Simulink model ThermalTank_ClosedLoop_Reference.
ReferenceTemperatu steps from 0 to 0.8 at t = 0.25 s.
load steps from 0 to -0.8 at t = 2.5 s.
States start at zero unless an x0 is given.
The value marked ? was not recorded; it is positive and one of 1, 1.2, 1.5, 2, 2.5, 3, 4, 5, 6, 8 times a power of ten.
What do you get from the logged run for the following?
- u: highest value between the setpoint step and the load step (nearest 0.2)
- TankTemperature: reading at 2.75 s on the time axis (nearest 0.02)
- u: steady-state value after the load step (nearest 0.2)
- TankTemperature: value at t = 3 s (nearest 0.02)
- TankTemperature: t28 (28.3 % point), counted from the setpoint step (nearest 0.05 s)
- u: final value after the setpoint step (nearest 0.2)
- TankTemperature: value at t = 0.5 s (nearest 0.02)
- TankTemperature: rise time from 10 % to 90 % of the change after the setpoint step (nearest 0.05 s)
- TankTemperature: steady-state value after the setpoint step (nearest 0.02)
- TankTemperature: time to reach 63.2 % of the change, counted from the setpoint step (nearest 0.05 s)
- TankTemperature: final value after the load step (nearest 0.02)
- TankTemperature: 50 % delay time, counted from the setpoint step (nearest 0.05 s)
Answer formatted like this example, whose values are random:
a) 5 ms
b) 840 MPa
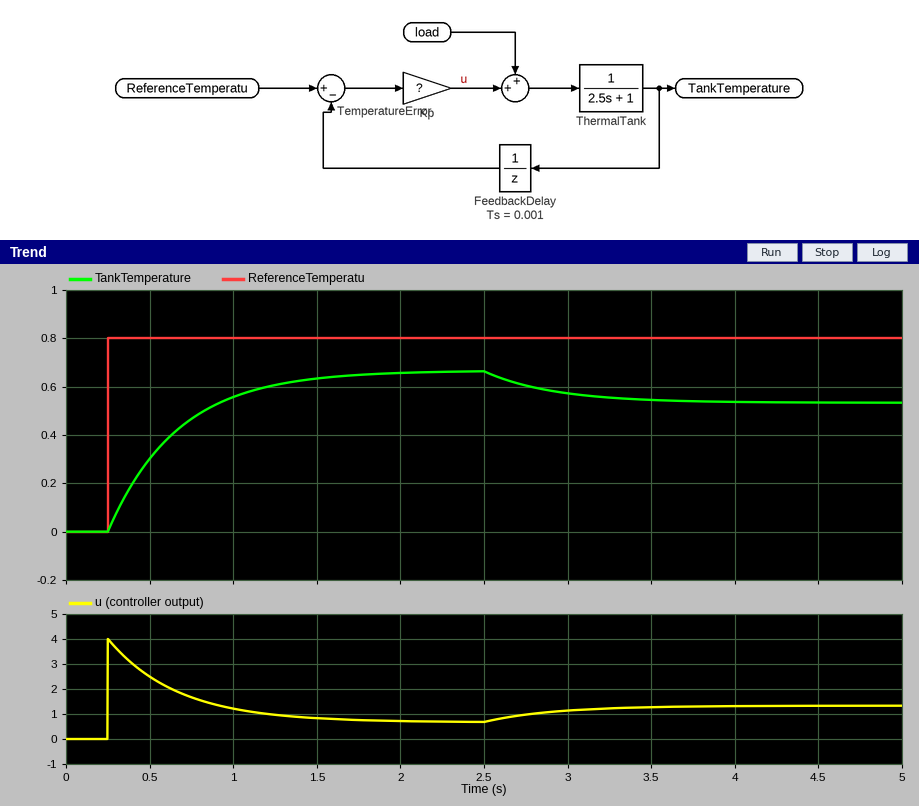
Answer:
a) 4.0
b) 0.60
c) 1.4
d) 0.58
e) 0.15 s
f) 0.6
g) 0.30
h) 0.90 s
i) 0.66
j) 0.40 s
k) 0.54
l) 0.30 s
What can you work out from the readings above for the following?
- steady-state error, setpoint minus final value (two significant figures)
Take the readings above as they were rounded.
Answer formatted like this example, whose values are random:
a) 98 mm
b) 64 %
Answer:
a) 0.14
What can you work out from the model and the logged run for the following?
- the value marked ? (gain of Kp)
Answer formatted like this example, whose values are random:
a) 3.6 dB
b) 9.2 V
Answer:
a) 5
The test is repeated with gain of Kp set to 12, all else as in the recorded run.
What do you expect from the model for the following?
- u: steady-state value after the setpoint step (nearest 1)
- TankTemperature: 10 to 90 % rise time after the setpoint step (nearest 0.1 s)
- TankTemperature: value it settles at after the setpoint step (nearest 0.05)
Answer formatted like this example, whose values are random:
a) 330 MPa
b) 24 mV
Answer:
a) 1
b) 0.4 s
c) 0.75
